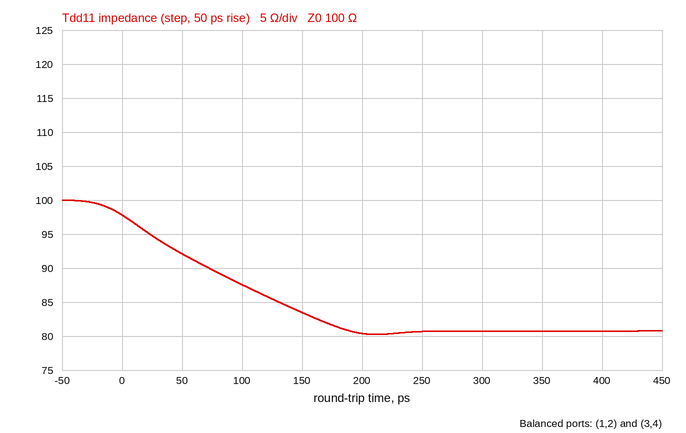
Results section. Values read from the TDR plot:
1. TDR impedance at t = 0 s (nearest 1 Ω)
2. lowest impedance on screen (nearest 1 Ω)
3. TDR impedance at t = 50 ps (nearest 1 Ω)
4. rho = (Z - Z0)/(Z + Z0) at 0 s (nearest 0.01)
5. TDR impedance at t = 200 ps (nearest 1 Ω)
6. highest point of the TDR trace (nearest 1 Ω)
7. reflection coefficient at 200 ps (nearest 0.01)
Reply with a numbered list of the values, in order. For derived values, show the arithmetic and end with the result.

1. 98 Ω
2. 80 Ω
3. 92 Ω
4. (98 − 100)/(98 + 100) ≈ -0.01
5. 80 Ω
6. 100 Ω
7. (80 − 100)/(80 + 100) ≈ -0.11
